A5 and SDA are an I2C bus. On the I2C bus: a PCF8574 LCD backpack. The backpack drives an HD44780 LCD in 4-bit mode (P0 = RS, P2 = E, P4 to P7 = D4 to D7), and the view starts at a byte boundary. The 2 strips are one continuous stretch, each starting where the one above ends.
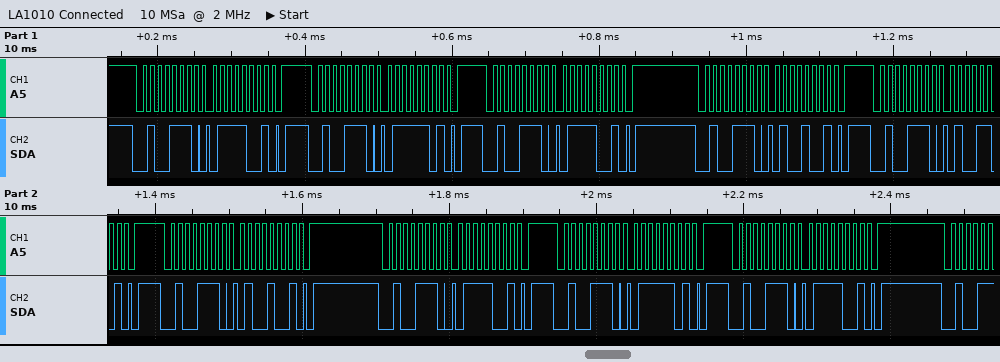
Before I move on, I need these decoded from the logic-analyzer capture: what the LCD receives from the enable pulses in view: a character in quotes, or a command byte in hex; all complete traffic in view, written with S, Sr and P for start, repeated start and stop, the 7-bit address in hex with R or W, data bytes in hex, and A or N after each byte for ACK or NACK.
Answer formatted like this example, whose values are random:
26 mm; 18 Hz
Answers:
't'; S 27W A 79 A P S 27W A 7D A P S 27W A 79 A P S 27W A 49 A P S 27W A 4D A P S 27W A 49 A P S 27W A 79 A P S 27W A 7D A P S 27W A 79 A P
